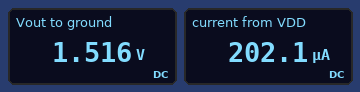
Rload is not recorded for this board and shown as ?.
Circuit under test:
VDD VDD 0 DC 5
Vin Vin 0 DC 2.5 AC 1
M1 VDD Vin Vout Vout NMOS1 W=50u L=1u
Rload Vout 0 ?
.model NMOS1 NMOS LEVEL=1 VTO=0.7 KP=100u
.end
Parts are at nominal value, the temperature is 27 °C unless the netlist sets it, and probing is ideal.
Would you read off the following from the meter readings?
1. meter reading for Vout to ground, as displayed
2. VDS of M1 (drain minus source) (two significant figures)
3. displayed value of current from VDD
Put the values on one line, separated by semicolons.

1.516 V; 3.5 V; 202.1 µA
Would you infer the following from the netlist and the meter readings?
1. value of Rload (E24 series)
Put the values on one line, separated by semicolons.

7.5 kΩ
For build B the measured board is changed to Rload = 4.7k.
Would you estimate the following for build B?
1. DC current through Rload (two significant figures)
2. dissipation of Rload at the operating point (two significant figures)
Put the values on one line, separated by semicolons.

310 µA; 450 µW
